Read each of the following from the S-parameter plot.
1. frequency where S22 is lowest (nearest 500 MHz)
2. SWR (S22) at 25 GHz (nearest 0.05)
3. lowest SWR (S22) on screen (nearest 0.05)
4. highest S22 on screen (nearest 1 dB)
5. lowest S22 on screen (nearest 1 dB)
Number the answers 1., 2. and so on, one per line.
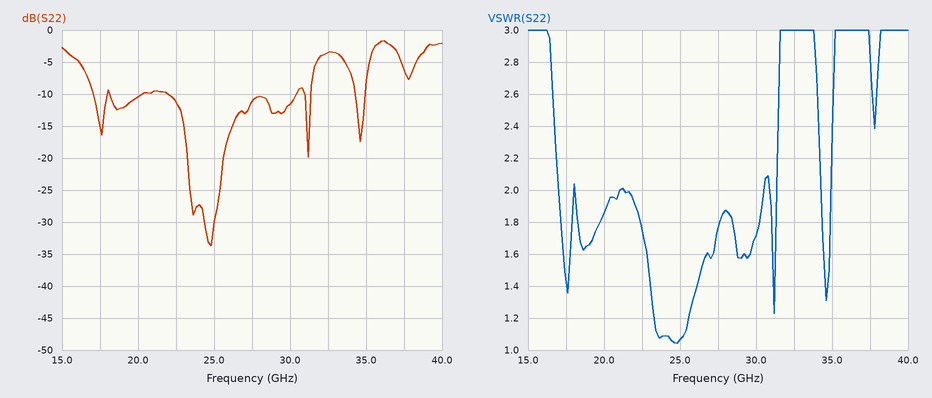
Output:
1. 25.0 GHz
2. 1.05
3. 1.05
4. -2 dB
5. -34 dB
